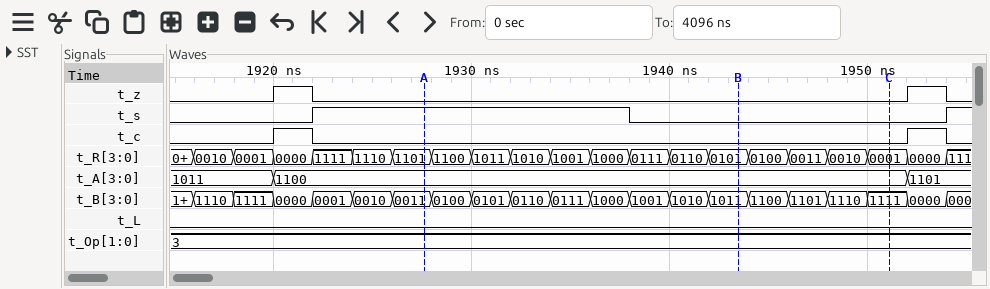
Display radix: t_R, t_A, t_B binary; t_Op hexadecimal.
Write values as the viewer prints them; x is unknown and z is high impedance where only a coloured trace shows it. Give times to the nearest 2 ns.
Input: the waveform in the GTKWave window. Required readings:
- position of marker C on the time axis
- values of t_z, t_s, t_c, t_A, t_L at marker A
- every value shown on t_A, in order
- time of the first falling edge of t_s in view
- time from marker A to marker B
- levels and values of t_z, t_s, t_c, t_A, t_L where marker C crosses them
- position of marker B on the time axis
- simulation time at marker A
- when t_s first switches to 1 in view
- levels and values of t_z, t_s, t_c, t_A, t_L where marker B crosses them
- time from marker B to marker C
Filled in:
1952 ns
t_z=0, t_s=1, t_c=0, t_A=1100, t_L=0
1011, 1100, 1101
1938 ns
16 ns
t_z=0, t_s=0, t_c=0, t_A=1100, t_L=0
1944 ns
1928 ns
1922 ns
t_z=0, t_s=0, t_c=0, t_A=1100, t_L=0
8 ns
